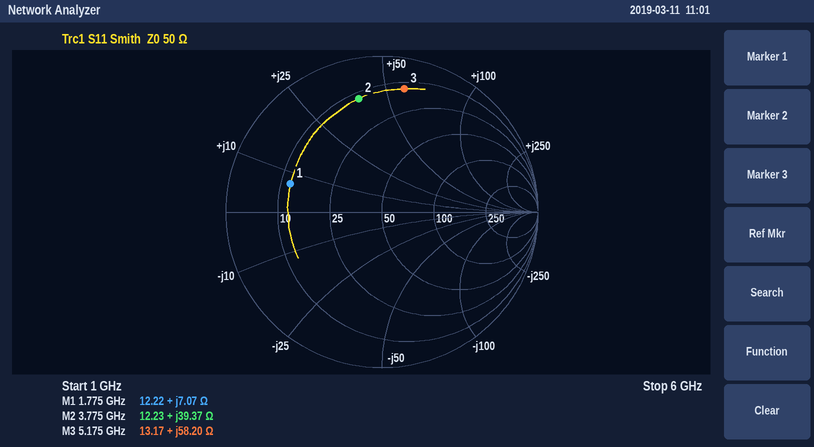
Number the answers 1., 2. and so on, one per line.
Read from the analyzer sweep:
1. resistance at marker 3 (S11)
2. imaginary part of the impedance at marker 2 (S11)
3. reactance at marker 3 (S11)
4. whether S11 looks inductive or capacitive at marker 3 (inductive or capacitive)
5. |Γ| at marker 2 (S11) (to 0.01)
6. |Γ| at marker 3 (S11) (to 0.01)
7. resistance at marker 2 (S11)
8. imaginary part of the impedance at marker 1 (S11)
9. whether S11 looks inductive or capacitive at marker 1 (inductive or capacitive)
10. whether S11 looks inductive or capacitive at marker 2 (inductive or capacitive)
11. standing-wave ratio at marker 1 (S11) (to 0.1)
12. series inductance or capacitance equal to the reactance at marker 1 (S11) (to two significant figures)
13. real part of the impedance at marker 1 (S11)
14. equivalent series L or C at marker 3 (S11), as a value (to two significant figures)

1. 13.17 Ω
2. +39.37 Ω
3. +58.20 Ω
4. inductive
5. 0.74
6. 0.80
7. 12.23 Ω
8. +7.07 Ω
9. inductive
10. inductive
11. 4.2
12. 630 pH
13. 12.22 Ω
14. 1.8 nH
